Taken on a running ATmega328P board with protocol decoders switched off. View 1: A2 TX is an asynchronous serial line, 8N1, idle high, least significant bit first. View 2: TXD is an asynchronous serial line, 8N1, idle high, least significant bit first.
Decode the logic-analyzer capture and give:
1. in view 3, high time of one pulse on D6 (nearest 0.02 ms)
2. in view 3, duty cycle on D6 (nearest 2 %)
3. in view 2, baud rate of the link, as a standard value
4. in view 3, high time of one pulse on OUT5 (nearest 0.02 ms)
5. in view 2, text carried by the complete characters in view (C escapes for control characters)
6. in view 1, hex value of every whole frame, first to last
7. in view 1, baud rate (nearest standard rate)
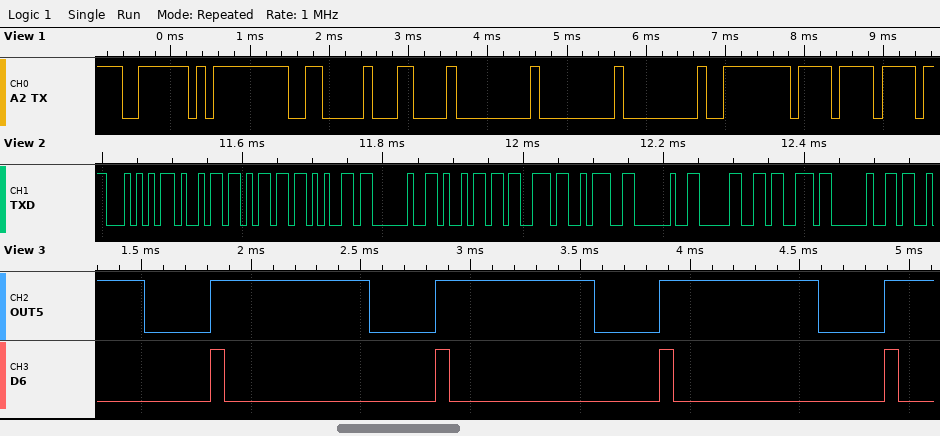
0.06 ms
6 %
115200 baud
0.72 ms
"Time is: 0s "
7E FF 06 0C 00 00 00 FE EF
9600 baud
